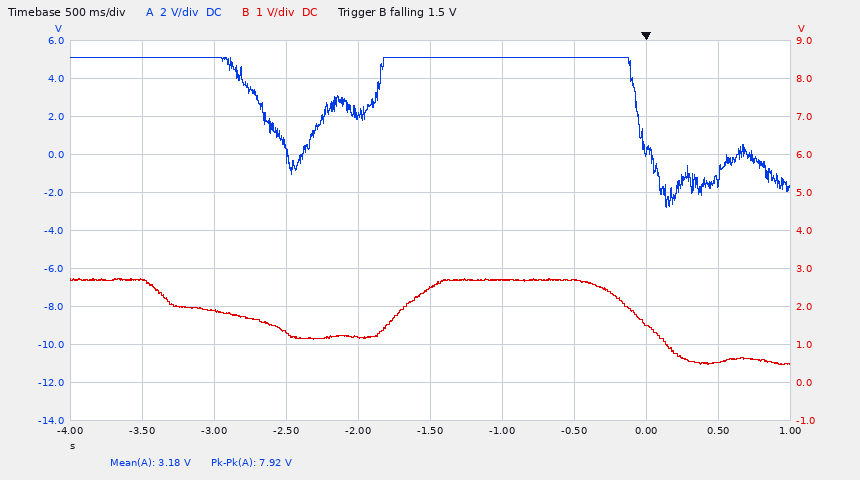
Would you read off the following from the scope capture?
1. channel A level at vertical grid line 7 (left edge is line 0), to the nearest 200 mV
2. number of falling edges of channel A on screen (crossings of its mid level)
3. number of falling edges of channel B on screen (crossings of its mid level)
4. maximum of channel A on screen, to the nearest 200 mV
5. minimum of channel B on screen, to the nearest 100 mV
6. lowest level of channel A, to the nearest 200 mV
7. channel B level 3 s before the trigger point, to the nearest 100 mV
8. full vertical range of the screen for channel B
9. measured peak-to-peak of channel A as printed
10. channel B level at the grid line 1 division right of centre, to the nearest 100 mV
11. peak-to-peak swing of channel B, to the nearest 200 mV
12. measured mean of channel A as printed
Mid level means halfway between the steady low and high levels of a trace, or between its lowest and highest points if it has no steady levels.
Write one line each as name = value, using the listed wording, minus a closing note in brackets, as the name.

channel A level at vertical grid line 7 (left edge is line 0), to the nearest 200 mV = 5.2 V
number of falling edges of channel A on screen = 2
number of falling edges of channel B on screen = 2
maximum of channel A on screen, to the nearest 200 mV = 5.2 V
minimum of channel B on screen, to the nearest 100 mV = 500 mV
lowest level of channel A, to the nearest 200 mV = -2.8 V
channel B level 3 s before the trigger point, to the nearest 100 mV = 1.9 V
full vertical range of the screen for channel B = 10 V
measured peak-to-peak of channel A as printed = 7.92 V
channel B level at the grid line 1 division right of centre, to the nearest 100 mV = 2.7 V
peak-to-peak swing of channel B, to the nearest 200 mV = 2.2 V
measured mean of channel A as printed = 3.18 V
